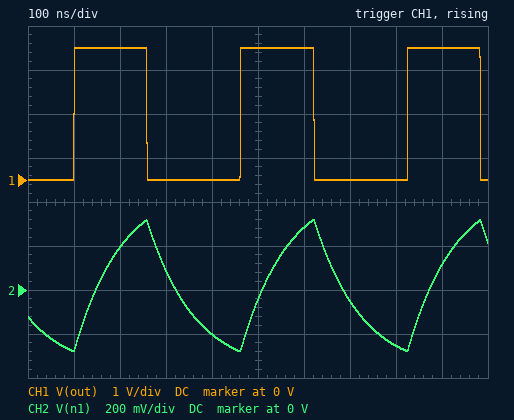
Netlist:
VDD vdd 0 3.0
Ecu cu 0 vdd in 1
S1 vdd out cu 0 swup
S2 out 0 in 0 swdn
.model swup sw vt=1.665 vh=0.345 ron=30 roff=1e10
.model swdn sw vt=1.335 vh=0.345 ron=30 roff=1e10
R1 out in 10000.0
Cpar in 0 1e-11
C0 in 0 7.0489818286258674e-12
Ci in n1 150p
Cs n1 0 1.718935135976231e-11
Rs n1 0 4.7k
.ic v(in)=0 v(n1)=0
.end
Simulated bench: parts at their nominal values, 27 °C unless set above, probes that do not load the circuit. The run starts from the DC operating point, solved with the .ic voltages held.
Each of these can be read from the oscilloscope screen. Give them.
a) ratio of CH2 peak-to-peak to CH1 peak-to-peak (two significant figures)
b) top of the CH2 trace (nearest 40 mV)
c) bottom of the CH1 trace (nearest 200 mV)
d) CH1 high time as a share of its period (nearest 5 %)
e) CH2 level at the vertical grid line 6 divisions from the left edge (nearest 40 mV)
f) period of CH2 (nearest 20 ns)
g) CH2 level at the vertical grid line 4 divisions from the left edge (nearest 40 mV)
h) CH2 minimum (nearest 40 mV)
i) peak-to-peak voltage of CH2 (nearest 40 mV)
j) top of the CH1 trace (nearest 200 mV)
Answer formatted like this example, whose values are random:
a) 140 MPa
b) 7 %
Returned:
a) 0.20
b) 320 mV
c) 0 V
d) 45 %
e) 280 mV
f) 360 ns
g) -200 mV
h) -280 mV
i) 600 mV
j) 3.0 V
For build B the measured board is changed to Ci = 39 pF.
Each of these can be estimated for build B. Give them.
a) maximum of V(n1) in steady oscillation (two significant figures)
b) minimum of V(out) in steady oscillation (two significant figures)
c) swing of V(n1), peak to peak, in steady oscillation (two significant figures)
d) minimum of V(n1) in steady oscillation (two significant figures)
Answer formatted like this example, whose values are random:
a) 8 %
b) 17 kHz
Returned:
a) 240 mV
b) 3.0 mV
c) 450 mV
d) -210 mV
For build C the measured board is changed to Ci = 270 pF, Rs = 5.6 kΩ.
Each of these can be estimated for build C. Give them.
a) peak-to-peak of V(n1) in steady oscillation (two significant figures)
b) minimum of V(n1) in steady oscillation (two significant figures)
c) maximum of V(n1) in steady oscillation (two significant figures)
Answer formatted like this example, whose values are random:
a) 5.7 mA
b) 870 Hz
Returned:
a) 640 mV
b) -300 mV
c) 340 mV
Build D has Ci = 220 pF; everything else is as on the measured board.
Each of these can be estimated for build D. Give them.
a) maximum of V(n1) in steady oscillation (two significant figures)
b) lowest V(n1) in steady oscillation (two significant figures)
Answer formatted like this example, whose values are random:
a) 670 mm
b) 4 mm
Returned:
a) 330 mV
b) -290 mV
